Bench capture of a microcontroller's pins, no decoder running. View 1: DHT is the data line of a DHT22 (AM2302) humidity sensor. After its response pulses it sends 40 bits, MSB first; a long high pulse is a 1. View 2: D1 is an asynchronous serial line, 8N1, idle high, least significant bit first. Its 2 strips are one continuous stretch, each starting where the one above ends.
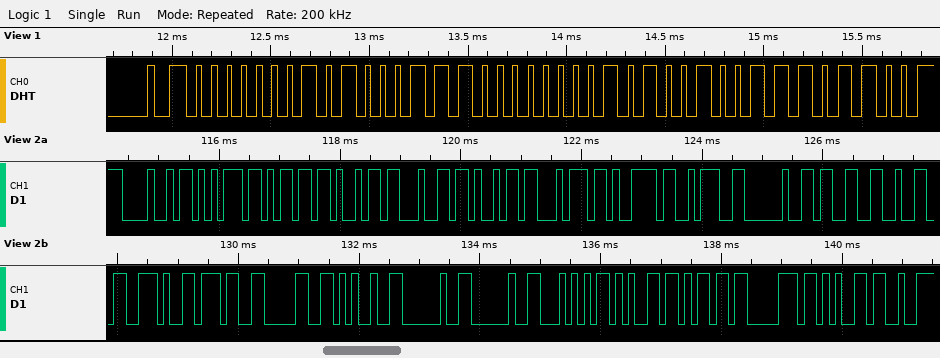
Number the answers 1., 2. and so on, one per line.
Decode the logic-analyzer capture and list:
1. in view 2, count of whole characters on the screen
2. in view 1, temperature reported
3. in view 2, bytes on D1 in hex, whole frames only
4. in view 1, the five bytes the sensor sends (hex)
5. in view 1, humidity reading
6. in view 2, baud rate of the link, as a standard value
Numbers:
1. 23
2. 16.4 °C
3. 48 75 6D 69 64 69 74 79 3A 20 33 32 2E 37 30 25 20 20 54 65 6D 70 65
4. 01 47 00 A4 EC
5. 32.7 %
6. 9600 baud
